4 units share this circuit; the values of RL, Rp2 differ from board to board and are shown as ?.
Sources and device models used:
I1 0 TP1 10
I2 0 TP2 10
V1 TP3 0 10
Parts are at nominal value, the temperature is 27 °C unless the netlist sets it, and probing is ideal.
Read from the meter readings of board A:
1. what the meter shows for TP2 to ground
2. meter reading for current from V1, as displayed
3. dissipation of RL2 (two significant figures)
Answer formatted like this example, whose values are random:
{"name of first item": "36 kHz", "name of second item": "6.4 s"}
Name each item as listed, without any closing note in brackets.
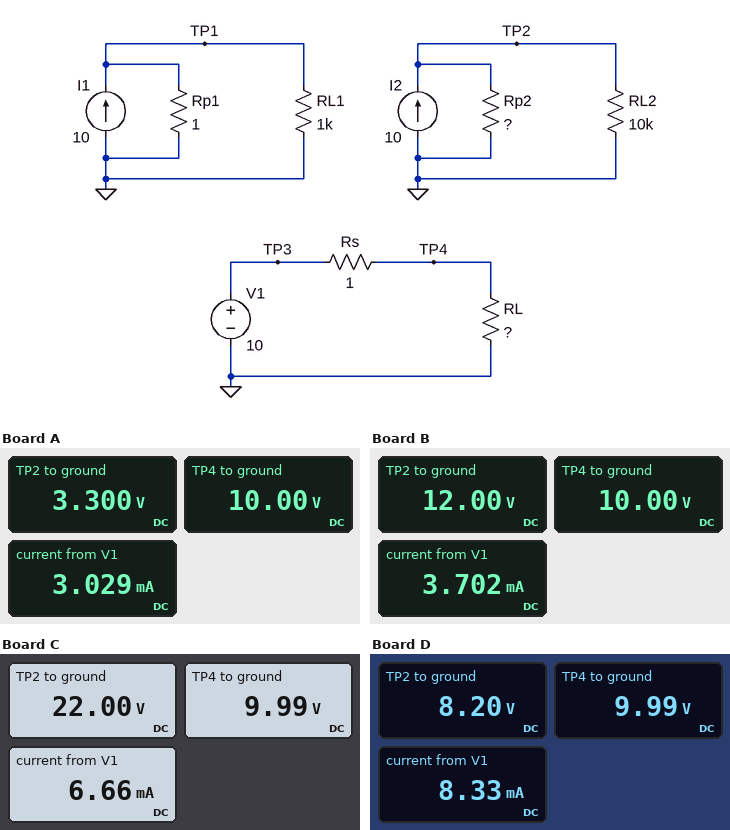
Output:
{"what the meter shows for TP2 to ground": "3.300 V", "meter reading for current from V1, as displayed": "3.029 mA", "dissipation of RL2": "1.1 mW"}
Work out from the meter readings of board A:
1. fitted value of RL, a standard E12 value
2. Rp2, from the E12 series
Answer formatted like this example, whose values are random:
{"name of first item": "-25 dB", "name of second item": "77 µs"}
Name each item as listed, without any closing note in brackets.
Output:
{"fitted value of RL, a standard E12 value": "3.3 kΩ", "Rp2, from the E12 series": "0.33 Ω"}
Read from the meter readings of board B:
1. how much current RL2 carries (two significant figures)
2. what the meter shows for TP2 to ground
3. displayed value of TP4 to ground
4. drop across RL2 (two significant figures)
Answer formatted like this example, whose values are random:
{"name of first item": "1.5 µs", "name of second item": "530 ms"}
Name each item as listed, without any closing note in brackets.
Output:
{"how much current RL2 carries": "1.2 mA", "what the meter shows for TP2 to ground": "12.00 V", "displayed value of TP4 to ground": "10.00 V", "drop across RL2": "12 V"}
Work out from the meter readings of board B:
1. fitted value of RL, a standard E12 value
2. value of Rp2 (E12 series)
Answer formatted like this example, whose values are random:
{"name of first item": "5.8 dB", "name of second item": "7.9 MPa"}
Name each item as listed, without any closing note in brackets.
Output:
{"fitted value of RL, a standard E12 value": "2.7 kΩ", "value of Rp2": "1.2 Ω"}
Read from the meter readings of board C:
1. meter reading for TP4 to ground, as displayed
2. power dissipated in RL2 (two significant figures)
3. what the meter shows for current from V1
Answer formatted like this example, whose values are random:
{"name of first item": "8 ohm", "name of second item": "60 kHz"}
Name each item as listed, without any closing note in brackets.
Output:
{"meter reading for TP4 to ground, as displayed": "9.99 V", "power dissipated in RL2": "48 mW", "what the meter shows for current from V1": "6.66 mA"}
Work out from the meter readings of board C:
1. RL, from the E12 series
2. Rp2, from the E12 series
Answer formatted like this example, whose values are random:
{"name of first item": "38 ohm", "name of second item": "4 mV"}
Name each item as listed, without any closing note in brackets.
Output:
{"RL, from the E12 series": "1.5 kΩ", "Rp2, from the E12 series": "2.2 Ω"}
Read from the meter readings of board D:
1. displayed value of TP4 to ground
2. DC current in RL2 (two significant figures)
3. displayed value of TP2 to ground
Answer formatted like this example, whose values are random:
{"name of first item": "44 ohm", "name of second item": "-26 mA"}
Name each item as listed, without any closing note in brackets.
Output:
{"displayed value of TP4 to ground": "9.99 V", "DC current in RL2": "820 µA", "displayed value of TP2 to ground": "8.20 V"}
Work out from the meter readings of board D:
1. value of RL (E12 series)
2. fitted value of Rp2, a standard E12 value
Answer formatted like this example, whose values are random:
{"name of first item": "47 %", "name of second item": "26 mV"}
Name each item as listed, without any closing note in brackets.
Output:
{"value of RL": "1.2 kΩ", "fitted value of Rp2, a standard E12 value": "0.82 Ω"}
